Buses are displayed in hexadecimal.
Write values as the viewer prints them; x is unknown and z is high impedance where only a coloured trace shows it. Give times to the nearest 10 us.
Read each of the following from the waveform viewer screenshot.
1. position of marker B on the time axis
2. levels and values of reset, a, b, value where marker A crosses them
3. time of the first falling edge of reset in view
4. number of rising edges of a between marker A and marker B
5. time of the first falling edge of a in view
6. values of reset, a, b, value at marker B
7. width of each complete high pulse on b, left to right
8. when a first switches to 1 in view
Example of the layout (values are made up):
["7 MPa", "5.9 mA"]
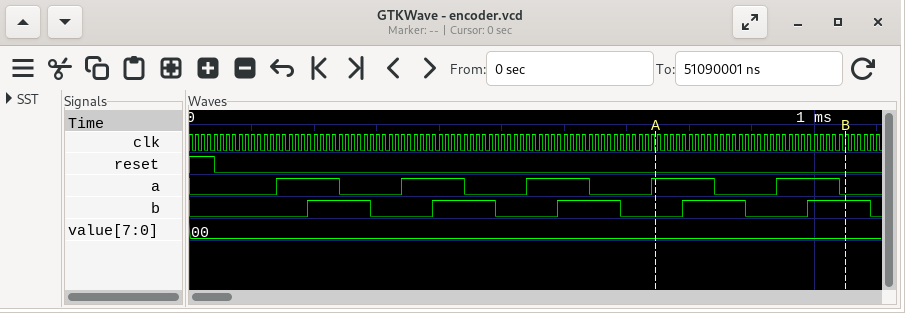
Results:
["1050 us", "reset=0, a=1, b=0, value=00", "40 us", "1", "240 us", "reset=0, a=0, b=1, value=00", "100 us, 100 us, 100 us, 100 us, 100 us", "140 us"]
